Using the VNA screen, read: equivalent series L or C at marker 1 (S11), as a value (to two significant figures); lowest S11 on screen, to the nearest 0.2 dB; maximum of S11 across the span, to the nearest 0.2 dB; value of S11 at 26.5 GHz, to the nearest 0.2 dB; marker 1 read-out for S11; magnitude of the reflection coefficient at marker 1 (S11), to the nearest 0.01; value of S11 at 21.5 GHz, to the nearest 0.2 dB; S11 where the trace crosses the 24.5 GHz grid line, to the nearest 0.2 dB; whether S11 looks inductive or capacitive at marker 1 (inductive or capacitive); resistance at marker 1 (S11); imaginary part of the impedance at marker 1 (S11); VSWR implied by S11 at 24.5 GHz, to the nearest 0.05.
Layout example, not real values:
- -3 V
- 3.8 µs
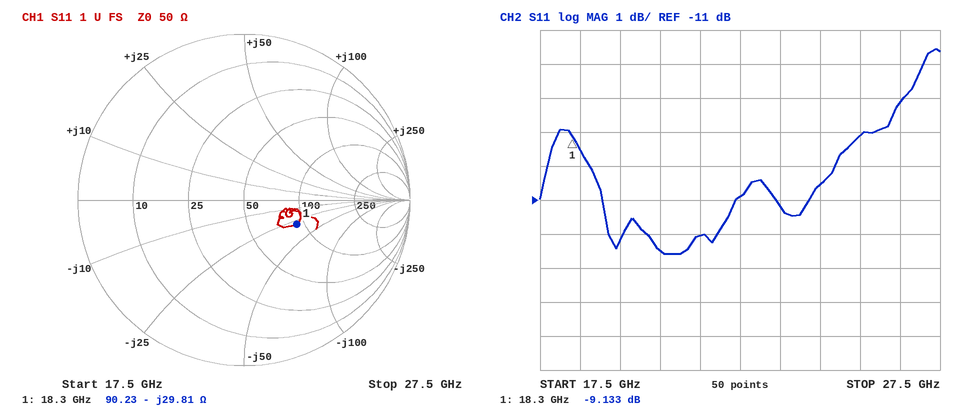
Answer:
- 290 fF
- -12.6 dB
- -6.6 dB
- -8.2 dB
- -9.133 dB
- 0.35
- -12.0 dB
- -10.6 dB
- capacitive
- 90.23 Ω
- -29.81 Ω
- 1.85
